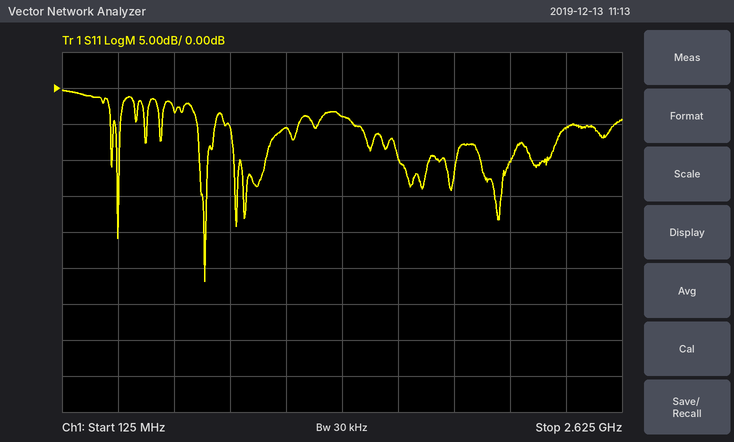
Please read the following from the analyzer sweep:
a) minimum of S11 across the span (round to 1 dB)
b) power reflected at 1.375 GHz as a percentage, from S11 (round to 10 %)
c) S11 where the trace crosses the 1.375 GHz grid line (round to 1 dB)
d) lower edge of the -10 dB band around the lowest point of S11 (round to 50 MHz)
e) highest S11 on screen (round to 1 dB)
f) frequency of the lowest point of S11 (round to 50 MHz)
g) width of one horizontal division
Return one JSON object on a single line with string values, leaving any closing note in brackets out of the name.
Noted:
{"minimum of S11 across the span": "-27 dB", "power reflected at 1.375 GHz as a percentage, from S11": "40 %", "S11 where the trace crosses the 1.375 GHz grid line": "-4 dB", "lower edge of the -10 dB band around the lowest point of S11": "750 MHz", "highest S11 on screen": "0 dB", "frequency of the lowest point of S11": "750 MHz", "width of one horizontal division": "250 MHz"}
